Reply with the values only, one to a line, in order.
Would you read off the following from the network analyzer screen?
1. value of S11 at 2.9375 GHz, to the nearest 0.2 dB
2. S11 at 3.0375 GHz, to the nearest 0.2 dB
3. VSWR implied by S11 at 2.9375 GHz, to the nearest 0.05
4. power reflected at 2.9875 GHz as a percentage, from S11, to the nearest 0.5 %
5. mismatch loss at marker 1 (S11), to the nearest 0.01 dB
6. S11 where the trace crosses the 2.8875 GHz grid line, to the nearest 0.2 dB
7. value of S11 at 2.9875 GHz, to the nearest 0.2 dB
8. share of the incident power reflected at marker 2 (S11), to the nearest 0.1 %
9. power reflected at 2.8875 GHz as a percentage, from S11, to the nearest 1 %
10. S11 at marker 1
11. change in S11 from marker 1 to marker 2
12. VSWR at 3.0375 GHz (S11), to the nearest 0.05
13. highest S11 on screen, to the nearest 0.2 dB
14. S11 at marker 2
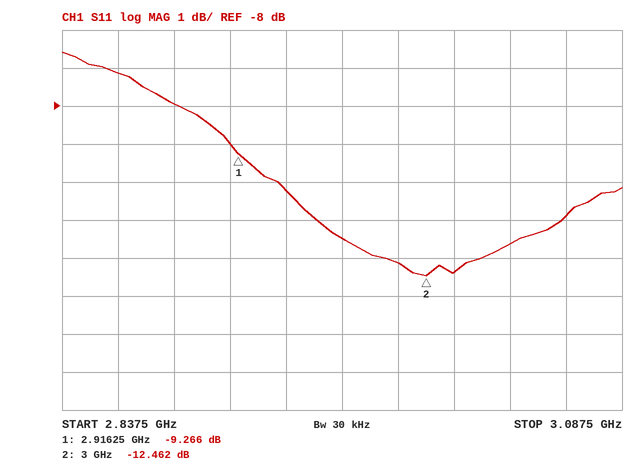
-10.2 dB
-11.6 dB
1.90
6.0 %
0.55 dB
-8.0 dB
-12.2 dB
5.7 %
16 %
-9.266 dB
-3.196 dB
1.70
-6.6 dB
-12.462 dB
